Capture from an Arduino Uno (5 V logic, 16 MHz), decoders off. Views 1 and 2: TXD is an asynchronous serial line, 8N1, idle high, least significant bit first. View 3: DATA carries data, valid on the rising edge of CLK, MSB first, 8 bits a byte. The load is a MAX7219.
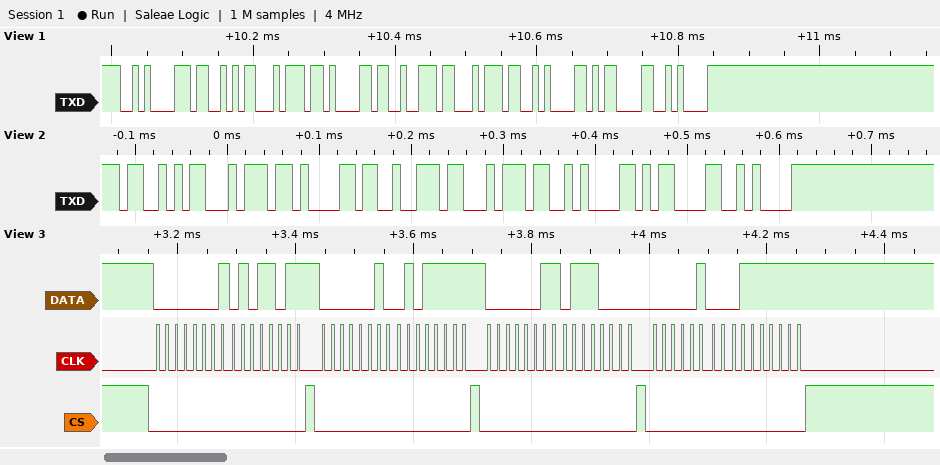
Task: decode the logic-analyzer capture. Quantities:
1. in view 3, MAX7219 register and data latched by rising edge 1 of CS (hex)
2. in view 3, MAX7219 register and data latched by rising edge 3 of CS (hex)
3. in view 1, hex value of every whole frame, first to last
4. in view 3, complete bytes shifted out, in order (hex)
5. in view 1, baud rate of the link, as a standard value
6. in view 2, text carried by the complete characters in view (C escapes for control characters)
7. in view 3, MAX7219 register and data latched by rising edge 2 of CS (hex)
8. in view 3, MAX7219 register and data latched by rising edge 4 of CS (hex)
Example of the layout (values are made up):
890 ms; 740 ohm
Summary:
register 0x1, data 0x5B; register 0x3, data 0x70; 0A 53 74 61 72 74 0A 0D 0A; 0x01 0x5B 0x02 0x5F 0x03 0x70 0x04 0x7F; 115200 baud; "Start\n\r\n"; register 0x2, data 0x5F; register 0x4, data 0x7F
